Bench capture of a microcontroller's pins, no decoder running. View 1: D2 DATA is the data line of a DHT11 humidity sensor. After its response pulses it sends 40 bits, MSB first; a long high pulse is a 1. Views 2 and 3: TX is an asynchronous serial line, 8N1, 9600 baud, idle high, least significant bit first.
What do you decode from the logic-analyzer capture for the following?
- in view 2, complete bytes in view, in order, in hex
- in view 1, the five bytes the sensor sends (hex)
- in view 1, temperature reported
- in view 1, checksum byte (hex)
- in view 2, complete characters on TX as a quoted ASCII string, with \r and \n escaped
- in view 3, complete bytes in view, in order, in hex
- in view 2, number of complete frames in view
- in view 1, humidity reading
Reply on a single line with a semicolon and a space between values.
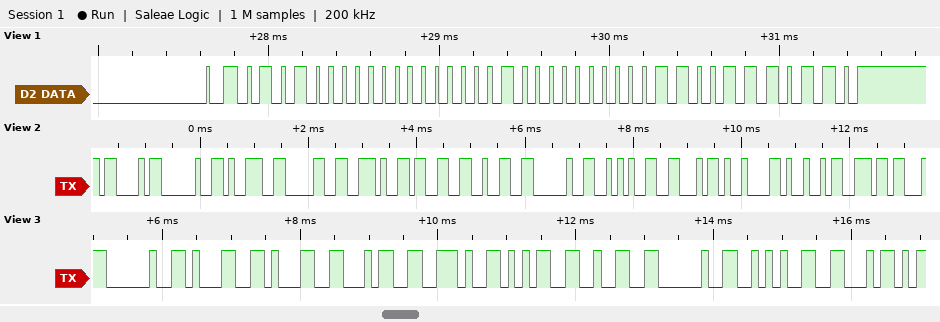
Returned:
0x43 0x20 0x39 0x30 0x2E 0x33 0x32 0x20 0x2A 0x46 0x09 0x49 0x6E; 50 00 20 06 76; 32.6 °C; 0x76; "C 90.32 *F\tIn"; 20 31 31 34 2E 35 32 20 2A 46; 13; 80 %
